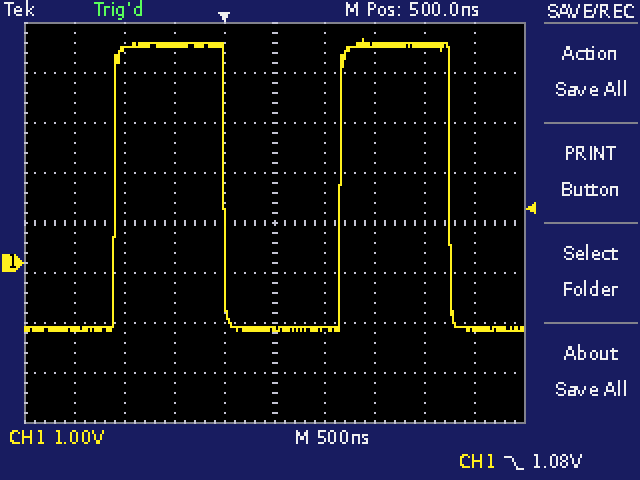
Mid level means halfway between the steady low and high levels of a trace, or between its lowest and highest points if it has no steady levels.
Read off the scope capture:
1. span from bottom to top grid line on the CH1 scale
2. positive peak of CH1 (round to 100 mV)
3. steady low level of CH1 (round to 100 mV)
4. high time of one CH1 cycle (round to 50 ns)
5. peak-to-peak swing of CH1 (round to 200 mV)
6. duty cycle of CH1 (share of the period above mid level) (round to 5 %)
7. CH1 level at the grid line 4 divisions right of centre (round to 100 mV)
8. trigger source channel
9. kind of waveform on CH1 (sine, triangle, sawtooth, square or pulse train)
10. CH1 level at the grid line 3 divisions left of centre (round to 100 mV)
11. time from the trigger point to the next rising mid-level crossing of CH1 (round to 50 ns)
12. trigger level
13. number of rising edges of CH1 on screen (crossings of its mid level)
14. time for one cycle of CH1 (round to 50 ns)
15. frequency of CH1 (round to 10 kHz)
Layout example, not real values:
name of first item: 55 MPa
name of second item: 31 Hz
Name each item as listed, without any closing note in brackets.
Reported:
span from bottom to top grid line on the CH1 scale: 8 V
positive peak of CH1: 4.5 V
steady low level of CH1: -1.3 V
high time of one CH1 cycle: 1.10 µs
peak-to-peak swing of CH1: 5.8 V
duty cycle of CH1 (share of the period above mid level): 50 %
CH1 level at the grid line 4 divisions right of centre: -1.3 V
trigger source channel: CH1
kind of waveform on CH1: square
CH1 level at the grid line 3 divisions left of centre: 4.3 V
time from the trigger point to the next rising mid-level crossing of CH1: 1.15 µs
trigger level: 1.08 V
number of rising edges of CH1 on screen: 2
time for one cycle of CH1: 2.25 µs
frequency of CH1: 440 kHz
